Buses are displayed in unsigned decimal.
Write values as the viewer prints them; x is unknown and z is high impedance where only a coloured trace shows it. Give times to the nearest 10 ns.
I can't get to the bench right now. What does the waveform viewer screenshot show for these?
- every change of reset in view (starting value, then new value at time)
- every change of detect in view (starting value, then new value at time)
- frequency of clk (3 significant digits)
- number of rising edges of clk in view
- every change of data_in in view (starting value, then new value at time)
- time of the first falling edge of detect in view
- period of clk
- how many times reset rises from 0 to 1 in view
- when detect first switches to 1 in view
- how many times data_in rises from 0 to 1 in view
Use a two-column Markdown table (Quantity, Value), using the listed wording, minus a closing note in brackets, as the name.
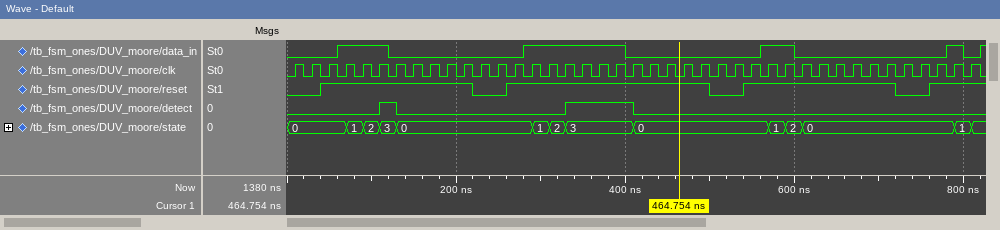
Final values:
| Quantity | Value |
|---|---|
| every change of reset in view | 0, 1 at 40 ns, 0 at 220 ns, 1 at 260 ns, 0 at 500 ns, 1 at 540 ns, 0 at 720 ns, 1 at 760 ns |
| every change of detect in view | 0, 1 at 110 ns, 0 at 130 ns, 1 at 330 ns, 0 at 410 ns |
| frequency of clk | 50.0 MHz |
| number of rising edges of clk in view | 41 |
| every change of data_in in view | 0, 1 at 60 ns, 0 at 120 ns, 1 at 280 ns, 0 at 400 ns, 1 at 560 ns, 0 at 600 ns, 1 at 780 ns, 0 at 800 ns, 1 at 820 ns |
| time of the first falling edge of detect in view | 130 ns |
| period of clk | 20 ns |
| how many times reset rises from 0 to 1 in view | 4 |
| when detect first switches to 1 in view | 110 ns |
| how many times data_in rises from 0 to 1 in view | 5 |
